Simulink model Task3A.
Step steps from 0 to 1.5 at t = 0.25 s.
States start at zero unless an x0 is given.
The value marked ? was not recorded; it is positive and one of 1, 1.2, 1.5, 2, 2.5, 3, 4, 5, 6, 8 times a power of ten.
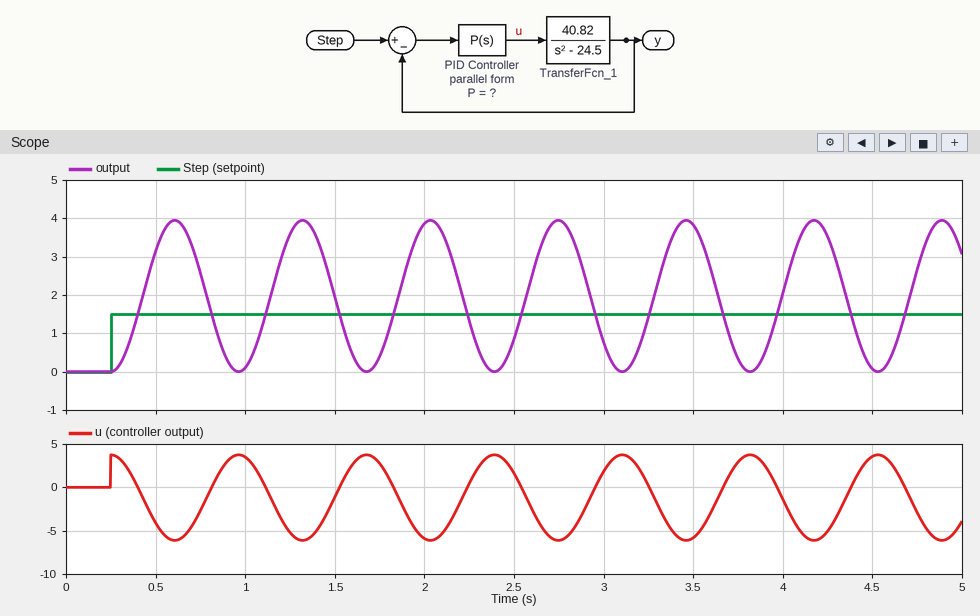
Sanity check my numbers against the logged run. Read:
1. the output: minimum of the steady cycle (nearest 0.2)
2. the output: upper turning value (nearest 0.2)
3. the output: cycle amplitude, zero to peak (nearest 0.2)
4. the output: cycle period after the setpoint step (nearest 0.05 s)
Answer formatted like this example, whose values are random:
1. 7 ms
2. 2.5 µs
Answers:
1. 0.0
2. 4.0
3. 2.0
4. 0.70 s
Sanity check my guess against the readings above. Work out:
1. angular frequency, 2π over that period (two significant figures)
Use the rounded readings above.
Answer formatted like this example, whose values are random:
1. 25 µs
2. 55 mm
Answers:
1. 9.0 rad/s
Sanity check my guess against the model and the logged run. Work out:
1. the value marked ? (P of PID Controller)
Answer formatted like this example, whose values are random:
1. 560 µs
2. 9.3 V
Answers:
1. 2.5
